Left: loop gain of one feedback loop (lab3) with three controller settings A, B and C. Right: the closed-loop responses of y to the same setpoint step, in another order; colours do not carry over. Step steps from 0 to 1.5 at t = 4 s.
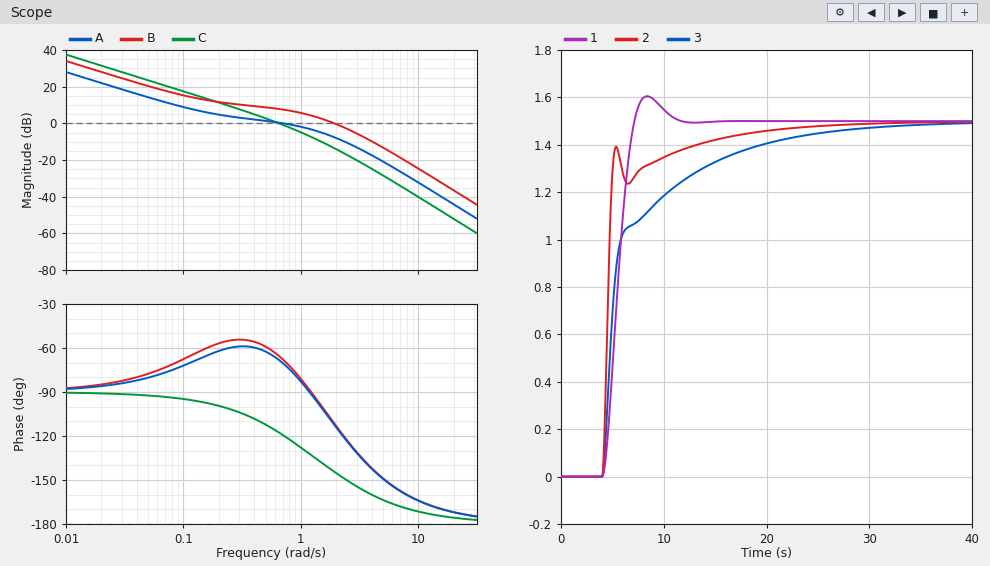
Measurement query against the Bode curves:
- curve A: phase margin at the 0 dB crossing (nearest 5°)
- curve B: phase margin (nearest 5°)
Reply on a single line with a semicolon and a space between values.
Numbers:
110°; 70°
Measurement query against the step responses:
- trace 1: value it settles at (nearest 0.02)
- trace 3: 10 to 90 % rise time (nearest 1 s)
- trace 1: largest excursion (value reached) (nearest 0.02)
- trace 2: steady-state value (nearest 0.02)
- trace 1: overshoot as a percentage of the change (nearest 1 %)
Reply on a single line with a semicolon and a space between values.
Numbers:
1.50; 12 s; 1.60; 1.50; 7 %
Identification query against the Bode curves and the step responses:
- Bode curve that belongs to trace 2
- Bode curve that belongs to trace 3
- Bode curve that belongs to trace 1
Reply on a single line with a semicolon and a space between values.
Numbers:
B; A; C
